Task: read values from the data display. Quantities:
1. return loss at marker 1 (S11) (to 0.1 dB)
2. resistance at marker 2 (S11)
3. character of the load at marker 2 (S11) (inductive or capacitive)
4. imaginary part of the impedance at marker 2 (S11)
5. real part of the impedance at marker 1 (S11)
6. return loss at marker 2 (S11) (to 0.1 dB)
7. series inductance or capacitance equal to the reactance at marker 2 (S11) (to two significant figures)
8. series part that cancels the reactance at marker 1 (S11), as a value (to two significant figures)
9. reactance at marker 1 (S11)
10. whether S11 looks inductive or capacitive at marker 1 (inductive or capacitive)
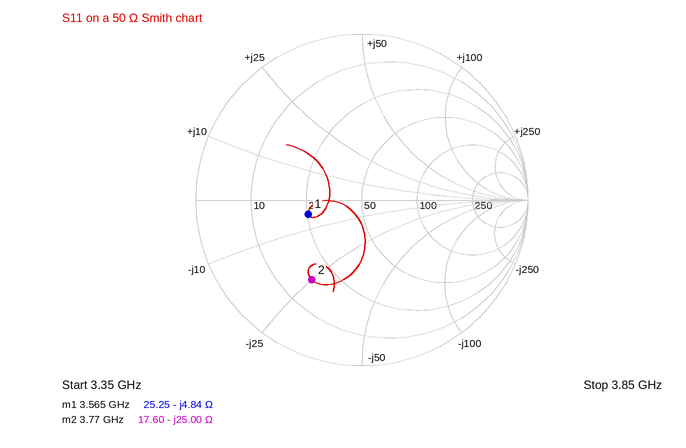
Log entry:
9.5 dB
17.60 Ω
capacitive
-25.00 Ω
25.25 Ω
4.9 dB
1.7 pF
220 pH
-4.84 Ω
capacitive
